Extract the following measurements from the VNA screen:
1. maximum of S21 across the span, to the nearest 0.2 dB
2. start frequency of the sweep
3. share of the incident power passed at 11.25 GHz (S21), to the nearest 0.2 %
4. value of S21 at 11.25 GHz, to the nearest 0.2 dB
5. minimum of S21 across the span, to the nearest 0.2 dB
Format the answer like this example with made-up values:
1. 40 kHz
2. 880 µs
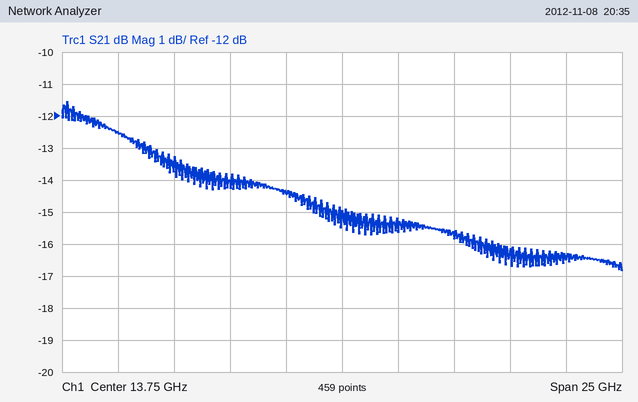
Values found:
1. -11.6 dB
2. 1.25 GHz
3. 3.6 %
4. -14.4 dB
5. -16.8 dB
